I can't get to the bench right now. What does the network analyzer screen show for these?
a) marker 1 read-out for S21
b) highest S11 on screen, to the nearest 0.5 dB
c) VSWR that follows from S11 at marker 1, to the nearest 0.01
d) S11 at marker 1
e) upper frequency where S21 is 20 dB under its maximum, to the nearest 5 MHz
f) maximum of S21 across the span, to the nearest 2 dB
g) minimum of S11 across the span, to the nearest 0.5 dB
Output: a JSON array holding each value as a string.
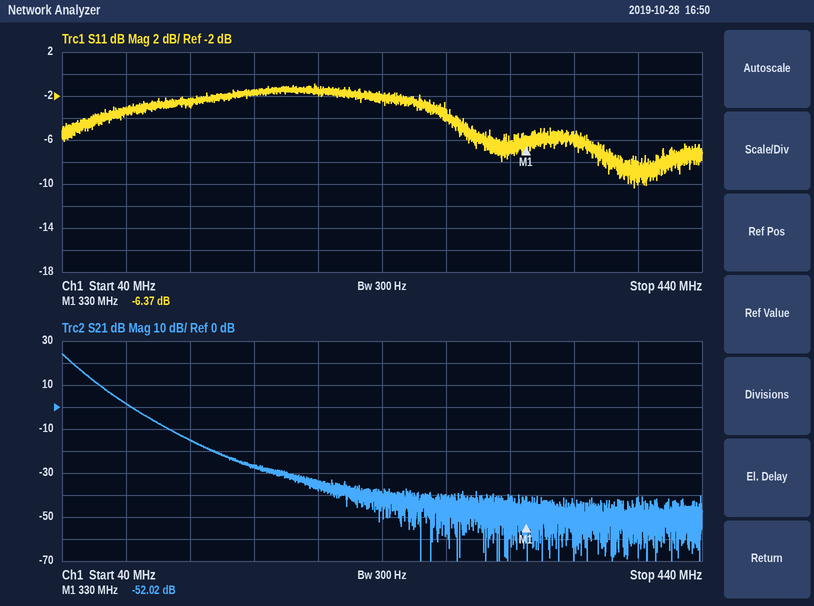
["-52.02 dB", "-1.0 dB", "2.85", "-6.37 dB", "75 MHz", "24 dB", "-10.5 dB"]
